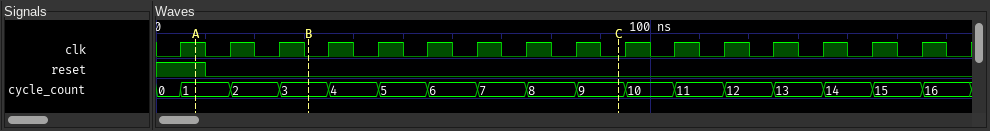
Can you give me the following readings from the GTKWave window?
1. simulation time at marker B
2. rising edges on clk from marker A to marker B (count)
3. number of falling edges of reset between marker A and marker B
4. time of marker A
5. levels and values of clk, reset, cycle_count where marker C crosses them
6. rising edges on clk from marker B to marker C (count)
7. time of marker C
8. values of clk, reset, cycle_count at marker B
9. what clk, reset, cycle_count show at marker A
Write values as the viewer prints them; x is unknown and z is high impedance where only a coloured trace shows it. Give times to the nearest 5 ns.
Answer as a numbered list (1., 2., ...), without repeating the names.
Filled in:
1. 30 ns
2. 2
3. 1
4. 10 ns
5. clk=0, reset=0, cycle_count=9
6. 6
7. 95 ns
8. clk=0, reset=0, cycle_count=3
9. clk=1, reset=1, cycle_count=1
